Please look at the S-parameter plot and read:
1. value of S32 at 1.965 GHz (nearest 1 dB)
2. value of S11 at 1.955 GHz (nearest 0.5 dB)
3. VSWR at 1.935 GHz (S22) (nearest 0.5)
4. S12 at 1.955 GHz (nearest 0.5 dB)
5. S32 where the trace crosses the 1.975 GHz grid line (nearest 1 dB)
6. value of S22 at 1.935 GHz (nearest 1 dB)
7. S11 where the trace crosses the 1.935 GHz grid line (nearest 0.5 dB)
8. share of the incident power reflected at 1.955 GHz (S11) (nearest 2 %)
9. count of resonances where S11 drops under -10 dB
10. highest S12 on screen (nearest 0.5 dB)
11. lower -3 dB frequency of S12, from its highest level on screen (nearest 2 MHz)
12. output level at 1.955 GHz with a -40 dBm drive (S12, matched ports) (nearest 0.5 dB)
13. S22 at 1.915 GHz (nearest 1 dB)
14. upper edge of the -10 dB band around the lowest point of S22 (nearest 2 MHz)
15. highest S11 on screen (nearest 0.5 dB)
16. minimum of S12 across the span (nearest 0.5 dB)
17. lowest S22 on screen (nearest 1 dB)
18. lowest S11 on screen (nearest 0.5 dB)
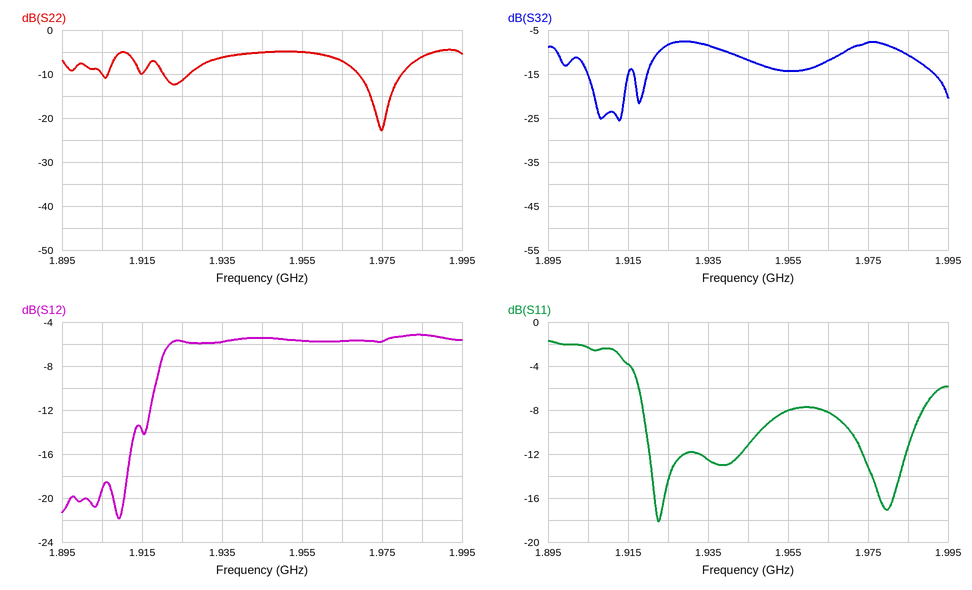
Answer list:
-12 dB
-8.0 dB
3.0
-5.5 dB
-8 dB
-6 dB
-12.5 dB
16 %
2
-5.0 dB
1.920 GHz
-45.5 dBm
-10 dB
1.980 GHz
-1.5 dB
-22.0 dB
-23 dB
-18.0 dB
